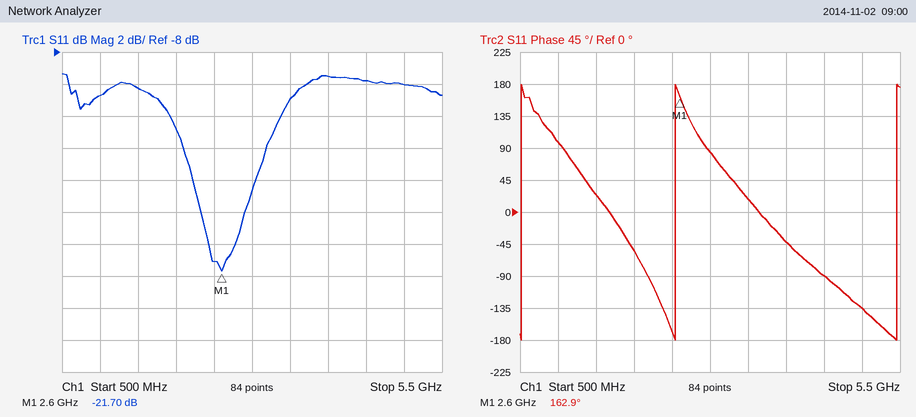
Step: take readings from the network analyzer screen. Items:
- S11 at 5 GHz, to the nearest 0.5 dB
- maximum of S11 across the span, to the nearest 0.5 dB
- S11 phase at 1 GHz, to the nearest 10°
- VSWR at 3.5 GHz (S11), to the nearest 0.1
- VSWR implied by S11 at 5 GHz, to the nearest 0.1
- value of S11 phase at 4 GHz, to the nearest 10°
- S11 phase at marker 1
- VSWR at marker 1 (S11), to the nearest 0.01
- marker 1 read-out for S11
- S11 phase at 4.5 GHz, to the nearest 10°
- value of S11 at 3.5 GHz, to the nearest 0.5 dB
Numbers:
-10.0 dB
-9.5 dB
100°
1.8
1.9
-40°
162.9°
1.18
-21.70 dB
-90°
-11.0 dB
